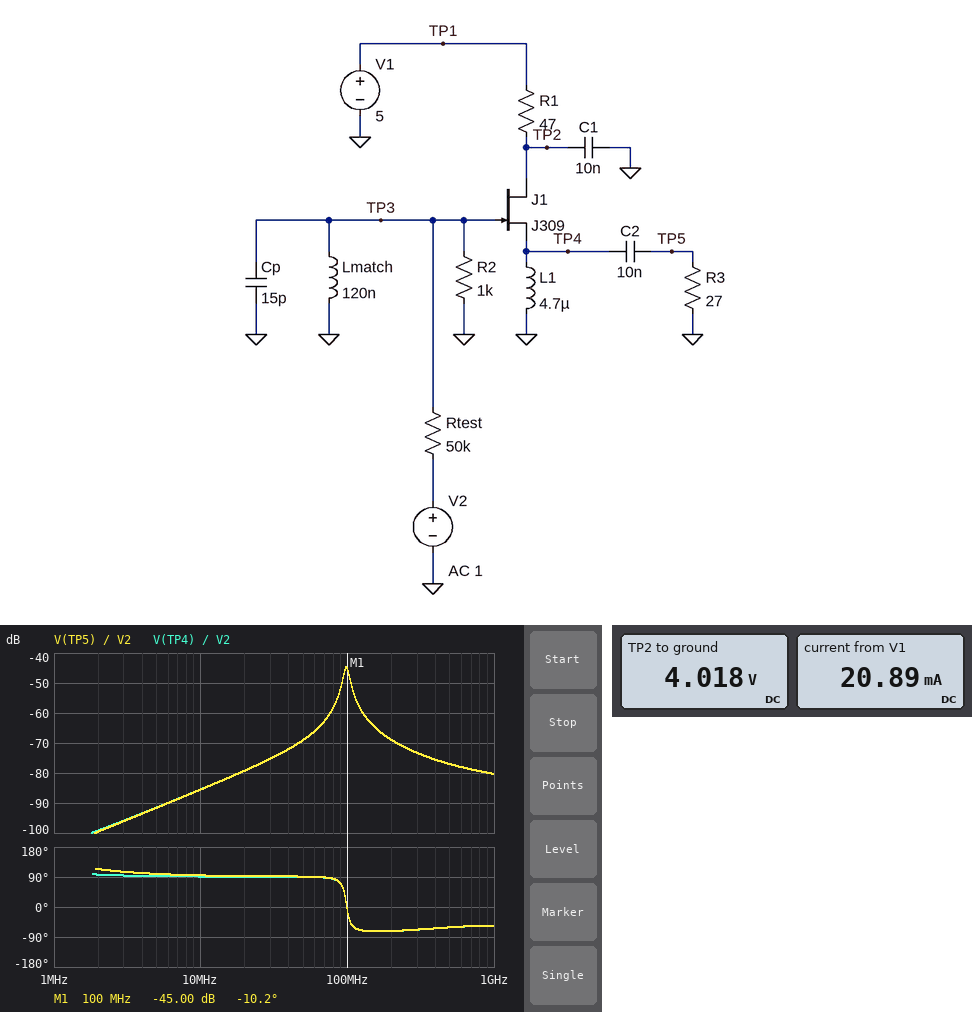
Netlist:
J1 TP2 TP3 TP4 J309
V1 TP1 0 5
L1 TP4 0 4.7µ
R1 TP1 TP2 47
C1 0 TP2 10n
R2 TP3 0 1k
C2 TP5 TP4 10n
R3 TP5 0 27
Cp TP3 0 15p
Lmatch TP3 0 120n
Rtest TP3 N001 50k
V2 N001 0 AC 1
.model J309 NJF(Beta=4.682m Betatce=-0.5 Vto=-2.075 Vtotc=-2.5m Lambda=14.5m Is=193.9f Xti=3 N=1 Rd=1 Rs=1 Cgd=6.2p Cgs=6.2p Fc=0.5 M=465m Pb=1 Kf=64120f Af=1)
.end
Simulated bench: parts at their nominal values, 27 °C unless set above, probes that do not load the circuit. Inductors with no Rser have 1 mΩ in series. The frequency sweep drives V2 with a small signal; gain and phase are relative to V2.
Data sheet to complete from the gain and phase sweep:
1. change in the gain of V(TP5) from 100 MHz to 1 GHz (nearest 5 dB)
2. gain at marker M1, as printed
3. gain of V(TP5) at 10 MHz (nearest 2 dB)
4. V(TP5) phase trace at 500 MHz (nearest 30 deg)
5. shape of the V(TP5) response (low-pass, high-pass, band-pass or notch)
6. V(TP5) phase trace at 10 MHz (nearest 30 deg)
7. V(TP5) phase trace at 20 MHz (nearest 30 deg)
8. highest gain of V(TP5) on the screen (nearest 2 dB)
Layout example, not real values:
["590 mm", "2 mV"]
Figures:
["-35 dB", "-45.00 dB", "-86 dB", "-60 deg", "band-pass", "90 deg", "90 deg", "-44 dB"]
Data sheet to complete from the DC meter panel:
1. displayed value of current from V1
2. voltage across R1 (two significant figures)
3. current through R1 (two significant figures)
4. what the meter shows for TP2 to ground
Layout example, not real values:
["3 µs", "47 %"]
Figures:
["20.89 mA", "980 mV", "21 mA", "4.018 V"]
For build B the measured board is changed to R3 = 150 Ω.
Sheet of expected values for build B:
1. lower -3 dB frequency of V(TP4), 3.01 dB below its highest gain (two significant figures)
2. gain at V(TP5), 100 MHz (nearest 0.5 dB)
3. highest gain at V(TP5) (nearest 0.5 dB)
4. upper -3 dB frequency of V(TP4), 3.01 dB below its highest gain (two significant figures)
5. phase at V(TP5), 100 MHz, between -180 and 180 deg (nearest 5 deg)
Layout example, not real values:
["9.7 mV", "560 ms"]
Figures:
["100 MHz", "-41.0 dB", "-38.0 dB", "110 MHz", "45 deg"]
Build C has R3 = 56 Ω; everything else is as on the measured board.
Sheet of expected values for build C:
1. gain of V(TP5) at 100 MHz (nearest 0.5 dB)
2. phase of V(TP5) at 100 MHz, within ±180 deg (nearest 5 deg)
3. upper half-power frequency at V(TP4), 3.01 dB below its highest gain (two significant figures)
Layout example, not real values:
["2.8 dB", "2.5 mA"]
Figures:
["-41.5 dB", "20 deg", "110 MHz"]
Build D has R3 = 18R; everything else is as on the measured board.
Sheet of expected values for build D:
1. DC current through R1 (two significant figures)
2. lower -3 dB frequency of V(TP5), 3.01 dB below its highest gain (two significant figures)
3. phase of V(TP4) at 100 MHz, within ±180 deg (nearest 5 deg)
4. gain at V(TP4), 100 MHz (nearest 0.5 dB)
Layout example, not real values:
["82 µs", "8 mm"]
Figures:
["21 mA", "93 MHz", "-25 deg", "-48.0 dB"]
